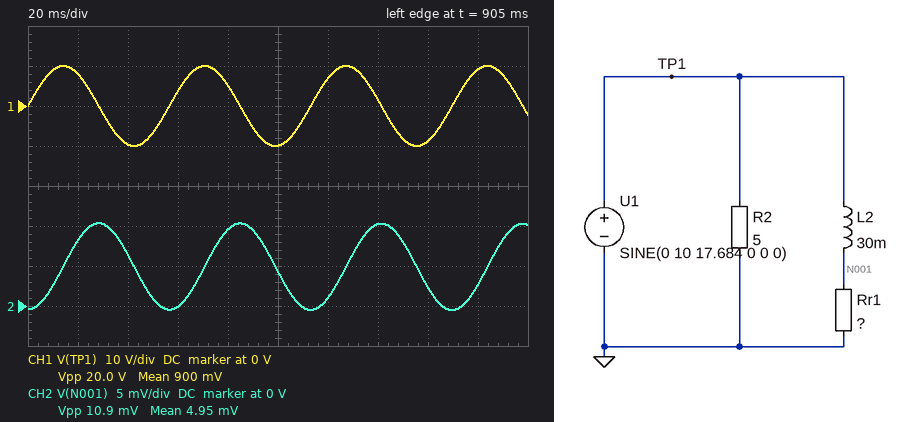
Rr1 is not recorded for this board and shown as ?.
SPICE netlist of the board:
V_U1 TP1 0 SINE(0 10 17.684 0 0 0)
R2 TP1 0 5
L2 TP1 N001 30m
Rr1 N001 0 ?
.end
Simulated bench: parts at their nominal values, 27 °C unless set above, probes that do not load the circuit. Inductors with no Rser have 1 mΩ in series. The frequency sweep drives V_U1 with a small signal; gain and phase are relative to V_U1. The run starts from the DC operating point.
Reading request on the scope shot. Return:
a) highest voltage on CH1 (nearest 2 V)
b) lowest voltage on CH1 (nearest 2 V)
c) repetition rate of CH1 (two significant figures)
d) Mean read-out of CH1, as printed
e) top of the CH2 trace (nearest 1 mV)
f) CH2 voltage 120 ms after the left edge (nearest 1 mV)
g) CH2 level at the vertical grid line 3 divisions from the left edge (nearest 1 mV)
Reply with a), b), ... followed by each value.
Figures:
a) 10 V
b) -10 V
c) 18 Hz
d) 900 mV
e) 10 mV
f) 1 mV
g) 0 V
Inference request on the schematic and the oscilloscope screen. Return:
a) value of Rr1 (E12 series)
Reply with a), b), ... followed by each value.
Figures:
a) 1.8 mΩ
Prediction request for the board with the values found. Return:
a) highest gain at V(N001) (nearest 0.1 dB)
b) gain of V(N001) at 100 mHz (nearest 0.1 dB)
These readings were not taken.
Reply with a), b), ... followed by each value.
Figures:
a) -3.8 dB
b) -20.5 dB
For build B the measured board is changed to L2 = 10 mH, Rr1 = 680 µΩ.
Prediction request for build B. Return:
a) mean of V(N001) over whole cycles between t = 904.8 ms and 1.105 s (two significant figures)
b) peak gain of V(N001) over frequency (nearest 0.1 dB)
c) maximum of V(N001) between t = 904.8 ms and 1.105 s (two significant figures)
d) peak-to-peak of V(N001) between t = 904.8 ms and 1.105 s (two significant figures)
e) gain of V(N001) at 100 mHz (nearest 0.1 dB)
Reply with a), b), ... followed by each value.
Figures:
a) 5.2 mV
b) -7.9 dB
c) 11 mV
d) 12 mV
e) -19.6 dB
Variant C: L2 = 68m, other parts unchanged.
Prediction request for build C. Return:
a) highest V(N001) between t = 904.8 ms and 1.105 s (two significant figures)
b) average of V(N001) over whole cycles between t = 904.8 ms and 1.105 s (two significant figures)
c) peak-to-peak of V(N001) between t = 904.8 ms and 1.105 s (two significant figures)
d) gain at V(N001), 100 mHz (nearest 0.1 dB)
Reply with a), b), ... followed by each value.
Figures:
a) 4.7 mV
b) 2.3 mV
c) 4.8 mV
d) -27.5 dB
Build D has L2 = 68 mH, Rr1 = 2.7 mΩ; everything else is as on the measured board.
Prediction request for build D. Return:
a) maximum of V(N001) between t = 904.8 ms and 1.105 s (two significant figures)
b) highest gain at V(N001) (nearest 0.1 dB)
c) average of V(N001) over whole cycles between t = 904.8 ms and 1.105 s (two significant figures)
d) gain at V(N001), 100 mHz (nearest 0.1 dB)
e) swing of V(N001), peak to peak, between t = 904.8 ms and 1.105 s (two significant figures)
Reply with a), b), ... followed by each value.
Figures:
a) 7.0 mV
b) -2.7 dB
c) 3.4 mV
d) -24.0 dB
e) 7.2 mV
